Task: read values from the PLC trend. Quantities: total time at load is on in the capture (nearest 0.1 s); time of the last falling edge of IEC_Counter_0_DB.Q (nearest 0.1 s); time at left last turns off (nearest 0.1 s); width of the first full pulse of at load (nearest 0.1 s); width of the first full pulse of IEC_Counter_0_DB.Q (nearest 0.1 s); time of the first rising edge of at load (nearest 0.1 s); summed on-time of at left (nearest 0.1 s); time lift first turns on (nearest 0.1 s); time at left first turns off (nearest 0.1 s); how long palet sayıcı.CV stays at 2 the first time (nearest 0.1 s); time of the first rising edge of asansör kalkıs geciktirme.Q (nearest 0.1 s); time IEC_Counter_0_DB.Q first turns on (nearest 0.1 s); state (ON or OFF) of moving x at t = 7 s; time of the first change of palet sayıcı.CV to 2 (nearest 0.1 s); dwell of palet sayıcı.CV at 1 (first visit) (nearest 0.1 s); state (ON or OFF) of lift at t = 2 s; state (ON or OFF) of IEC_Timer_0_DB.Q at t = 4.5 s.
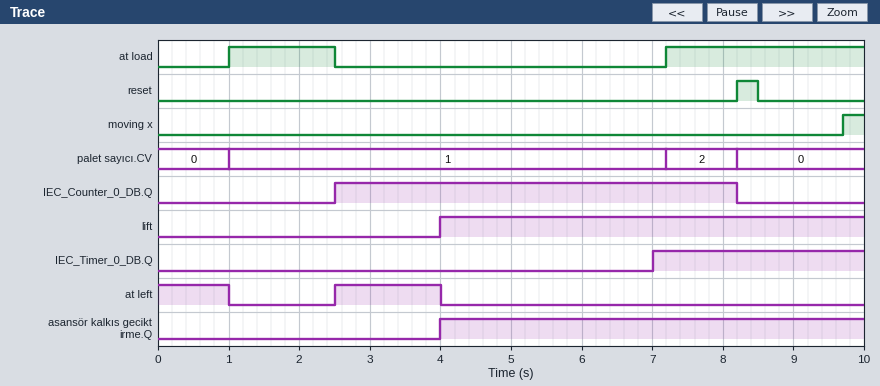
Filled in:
4.3 s
8.2 s
4.0 s
1.5 s
5.7 s
1.0 s
2.5 s
4.0 s
1.0 s
1.0 s
4.0 s
2.5 s
OFF
7.2 s
6.2 s
OFF
OFF
